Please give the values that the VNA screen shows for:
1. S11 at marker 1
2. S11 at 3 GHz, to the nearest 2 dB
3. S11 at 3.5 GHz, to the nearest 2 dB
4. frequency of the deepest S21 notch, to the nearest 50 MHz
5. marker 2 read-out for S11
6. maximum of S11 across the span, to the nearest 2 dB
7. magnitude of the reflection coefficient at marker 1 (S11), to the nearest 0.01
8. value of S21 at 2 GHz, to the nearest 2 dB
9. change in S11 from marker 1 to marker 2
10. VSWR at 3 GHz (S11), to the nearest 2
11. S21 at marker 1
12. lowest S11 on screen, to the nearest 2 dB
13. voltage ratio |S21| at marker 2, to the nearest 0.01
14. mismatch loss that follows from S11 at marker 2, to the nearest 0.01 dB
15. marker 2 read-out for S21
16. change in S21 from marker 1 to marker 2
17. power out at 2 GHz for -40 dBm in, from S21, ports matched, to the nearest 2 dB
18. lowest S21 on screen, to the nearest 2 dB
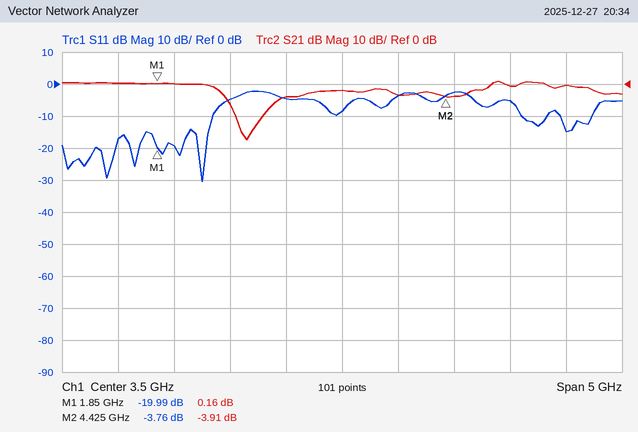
-19.99 dB
-4 dB
-8 dB
2.65 GHz
-3.76 dB
-2 dB
0.10
0 dB
16.23 dB
4
0.16 dB
-30 dB
0.64
2.37 dB
-3.91 dB
-4.07 dB
-40 dBm
-18 dB
